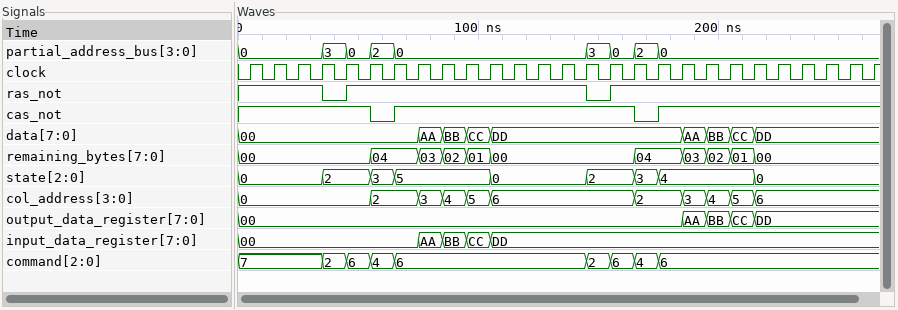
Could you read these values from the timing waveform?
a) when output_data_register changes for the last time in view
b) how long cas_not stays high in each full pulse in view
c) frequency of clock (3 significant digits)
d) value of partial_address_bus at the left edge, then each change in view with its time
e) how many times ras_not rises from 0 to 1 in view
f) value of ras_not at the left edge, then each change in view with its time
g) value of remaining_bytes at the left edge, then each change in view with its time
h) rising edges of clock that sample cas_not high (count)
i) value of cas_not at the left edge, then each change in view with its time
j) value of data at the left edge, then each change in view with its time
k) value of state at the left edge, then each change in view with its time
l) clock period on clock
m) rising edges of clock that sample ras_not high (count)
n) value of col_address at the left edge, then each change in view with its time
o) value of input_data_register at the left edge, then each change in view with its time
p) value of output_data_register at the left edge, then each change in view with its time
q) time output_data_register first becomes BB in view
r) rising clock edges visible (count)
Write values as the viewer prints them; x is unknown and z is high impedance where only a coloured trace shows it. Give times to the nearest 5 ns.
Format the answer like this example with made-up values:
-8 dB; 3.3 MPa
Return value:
215 ns; 100 ns; 100 MHz; 0, 3 at 35 ns, 0 at 45 ns, 2 at 55 ns, 0 at 65 ns, 3 at 145 ns, 0 at 155 ns, 2 at 165 ns, 0 at 175 ns; 2; 1, 0 at 35 ns, 1 at 45 ns, 0 at 145 ns, 1 at 155 ns; 00, 04 at 55 ns, 03 at 75 ns, 02 at 85 ns, 01 at 95 ns, 00 at 105 ns, 04 at 165 ns, 03 at 185 ns, 02 at 195 ns, 01 at 205 ns, 00 at 215 ns; 25; 1, 0 at 55 ns, 1 at 65 ns, 0 at 165 ns, 1 at 175 ns; 00, AA at 75 ns, BB at 85 ns, CC at 95 ns, DD at 105 ns, AA at 185 ns, BB at 195 ns, CC at 205 ns, DD at 215 ns; 0, 2 at 35 ns, 3 at 55 ns, 5 at 65 ns, 0 at 105 ns, 2 at 145 ns, 3 at 165 ns, 4 at 175 ns, 0 at 215 ns; 10 ns; 25; 0, 2 at 55 ns, 3 at 75 ns, 4 at 85 ns, 5 at 95 ns, 6 at 105 ns, 2 at 165 ns, 3 at 185 ns, 4 at 195 ns, 5 at 205 ns, 6 at 215 ns; 00, AA at 75 ns, BB at 85 ns, CC at 95 ns, DD at 105 ns; 00, AA at 185 ns, BB at 195 ns, CC at 205 ns, DD at 215 ns; 195 ns; 27
